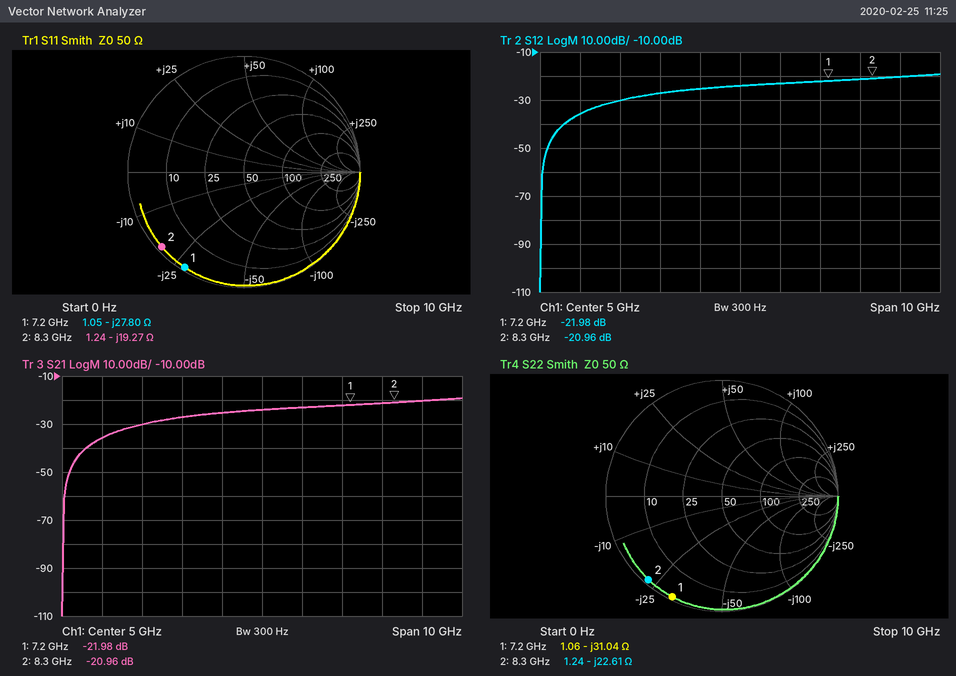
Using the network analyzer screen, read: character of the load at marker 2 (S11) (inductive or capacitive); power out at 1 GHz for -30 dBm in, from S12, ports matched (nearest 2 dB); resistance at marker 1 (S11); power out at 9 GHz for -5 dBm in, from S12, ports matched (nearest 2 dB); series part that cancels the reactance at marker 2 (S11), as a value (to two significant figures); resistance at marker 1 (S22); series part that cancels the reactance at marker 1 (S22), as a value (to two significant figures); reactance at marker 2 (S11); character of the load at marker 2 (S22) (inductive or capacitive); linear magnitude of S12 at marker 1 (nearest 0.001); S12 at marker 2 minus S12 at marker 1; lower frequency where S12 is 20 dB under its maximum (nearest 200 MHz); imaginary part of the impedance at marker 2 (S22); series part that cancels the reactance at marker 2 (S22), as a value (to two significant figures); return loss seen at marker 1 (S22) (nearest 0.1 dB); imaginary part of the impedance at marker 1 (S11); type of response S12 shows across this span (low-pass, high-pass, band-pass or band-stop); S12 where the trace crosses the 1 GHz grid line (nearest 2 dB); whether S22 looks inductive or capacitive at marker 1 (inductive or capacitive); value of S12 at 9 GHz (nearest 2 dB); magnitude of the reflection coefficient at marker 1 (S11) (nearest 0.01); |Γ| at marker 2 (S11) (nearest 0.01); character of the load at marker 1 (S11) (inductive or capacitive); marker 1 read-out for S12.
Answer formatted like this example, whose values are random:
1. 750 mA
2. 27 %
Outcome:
1. capacitive
2. -66 dBm
3. 1.05 Ω
4. -26 dBm
5. 370 pH
6. 1.06 Ω
7. 690 pH
8. -19.27 Ω
9. capacitive
10. 0.080
11. 1.02 dB
12. 600 MHz
13. -22.61 Ω
14. 430 pH
15. 0.3 dB
16. -27.80 Ω
17. high-pass
18. -36 dB
19. capacitive
20. -20 dB
21. 0.97
22. 0.96
23. capacitive
24. -21.98 dB
